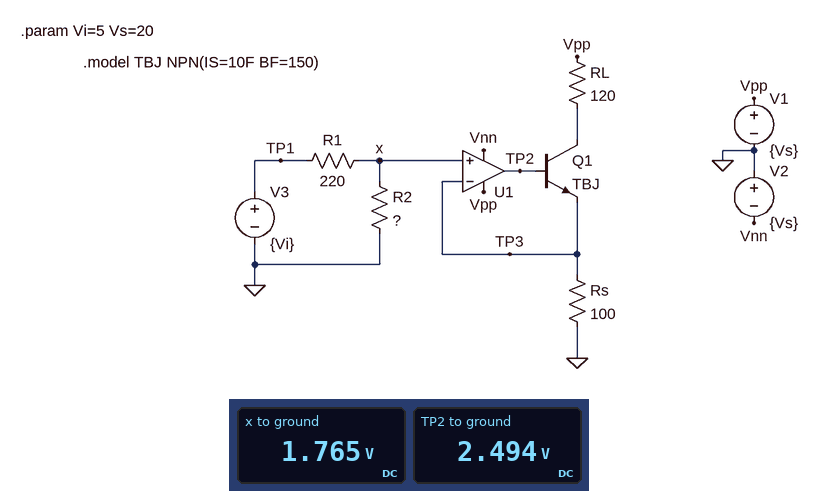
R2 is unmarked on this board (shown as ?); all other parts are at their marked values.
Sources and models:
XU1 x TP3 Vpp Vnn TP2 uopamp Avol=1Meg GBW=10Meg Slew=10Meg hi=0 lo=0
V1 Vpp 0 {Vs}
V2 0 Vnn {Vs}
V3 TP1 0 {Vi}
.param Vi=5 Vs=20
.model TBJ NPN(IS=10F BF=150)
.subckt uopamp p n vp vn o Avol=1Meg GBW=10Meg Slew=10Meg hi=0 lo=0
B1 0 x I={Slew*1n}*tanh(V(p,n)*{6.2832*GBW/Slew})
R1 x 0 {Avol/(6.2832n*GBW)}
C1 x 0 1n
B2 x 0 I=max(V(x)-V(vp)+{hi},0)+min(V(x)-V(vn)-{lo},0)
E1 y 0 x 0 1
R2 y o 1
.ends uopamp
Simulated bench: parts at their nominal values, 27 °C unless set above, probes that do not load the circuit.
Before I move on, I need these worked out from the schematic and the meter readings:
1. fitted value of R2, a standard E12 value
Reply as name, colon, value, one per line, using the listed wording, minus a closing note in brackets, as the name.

fitted value of R2, a standard E12 value: 120 Ω
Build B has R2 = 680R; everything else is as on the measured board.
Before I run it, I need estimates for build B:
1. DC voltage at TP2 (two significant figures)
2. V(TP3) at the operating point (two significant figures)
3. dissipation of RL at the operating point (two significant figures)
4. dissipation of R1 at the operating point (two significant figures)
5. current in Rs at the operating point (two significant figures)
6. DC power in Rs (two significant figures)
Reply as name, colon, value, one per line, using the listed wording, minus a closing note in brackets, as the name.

DC voltage at TP2: 4.5 V
V(TP3) at the operating point: 3.8 V
dissipation of RL at the operating point: 170 mW
dissipation of R1 at the operating point: 6.8 mW
current in Rs at the operating point: 38 mA
DC power in Rs: 140 mW
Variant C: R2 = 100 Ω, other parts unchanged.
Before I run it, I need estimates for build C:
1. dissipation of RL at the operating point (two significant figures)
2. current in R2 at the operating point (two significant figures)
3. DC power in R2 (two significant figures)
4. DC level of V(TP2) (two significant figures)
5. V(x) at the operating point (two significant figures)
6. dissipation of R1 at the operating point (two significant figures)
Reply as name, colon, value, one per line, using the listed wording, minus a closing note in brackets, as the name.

dissipation of RL at the operating point: 29 mW
current in R2 at the operating point: 16 mA
DC power in R2: 24 mW
DC level of V(TP2): 2.3 V
V(x) at the operating point: 1.6 V
dissipation of R1 at the operating point: 54 mW
